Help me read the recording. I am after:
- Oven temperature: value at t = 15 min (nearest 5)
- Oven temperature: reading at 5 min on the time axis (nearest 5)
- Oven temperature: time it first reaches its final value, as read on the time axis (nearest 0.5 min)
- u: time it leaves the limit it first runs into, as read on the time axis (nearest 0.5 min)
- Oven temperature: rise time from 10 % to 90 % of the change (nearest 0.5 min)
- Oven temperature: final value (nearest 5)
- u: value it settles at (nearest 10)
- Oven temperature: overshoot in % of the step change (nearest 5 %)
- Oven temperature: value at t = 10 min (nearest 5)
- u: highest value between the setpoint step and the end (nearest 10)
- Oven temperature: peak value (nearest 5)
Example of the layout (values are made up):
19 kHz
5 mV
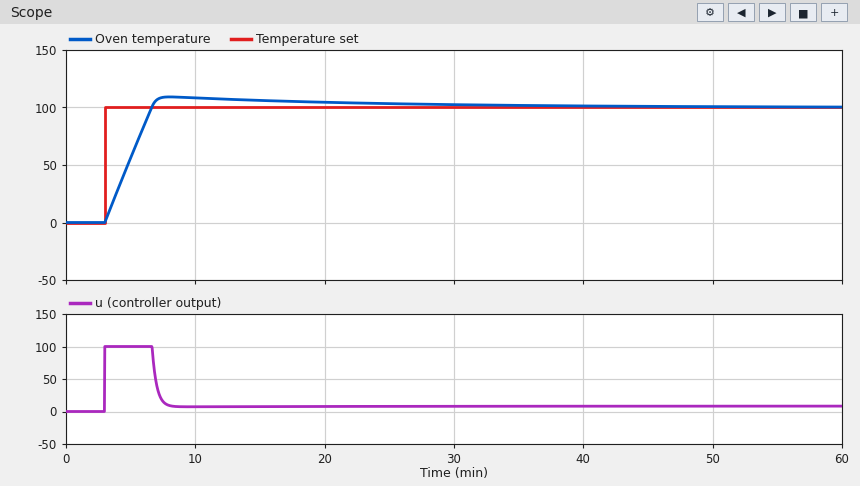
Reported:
105
55
6.5 min
6.5 min
3.0 min
100
10
10 %
110
100
110
